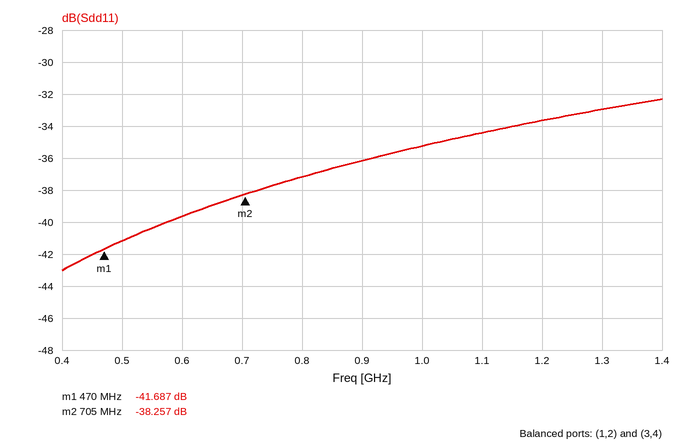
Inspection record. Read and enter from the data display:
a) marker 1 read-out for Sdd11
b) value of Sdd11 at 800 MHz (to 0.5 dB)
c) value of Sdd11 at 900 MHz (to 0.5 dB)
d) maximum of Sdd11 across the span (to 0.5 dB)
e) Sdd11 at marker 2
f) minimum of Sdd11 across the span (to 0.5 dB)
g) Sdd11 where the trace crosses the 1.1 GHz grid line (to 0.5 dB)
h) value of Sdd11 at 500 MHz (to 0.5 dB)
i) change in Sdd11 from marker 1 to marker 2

-41.687 dB
-37.0 dB
-36.0 dB
-32.5 dB
-38.257 dB
-43.0 dB
-34.5 dB
-41.0 dB
3.430 dB
